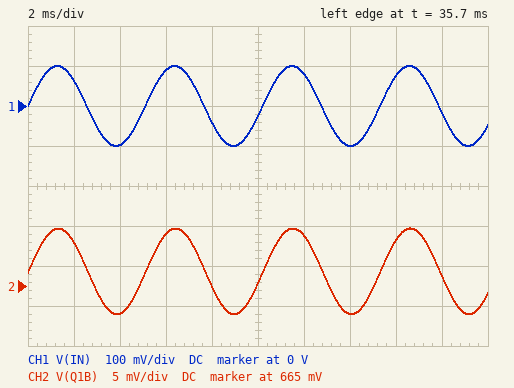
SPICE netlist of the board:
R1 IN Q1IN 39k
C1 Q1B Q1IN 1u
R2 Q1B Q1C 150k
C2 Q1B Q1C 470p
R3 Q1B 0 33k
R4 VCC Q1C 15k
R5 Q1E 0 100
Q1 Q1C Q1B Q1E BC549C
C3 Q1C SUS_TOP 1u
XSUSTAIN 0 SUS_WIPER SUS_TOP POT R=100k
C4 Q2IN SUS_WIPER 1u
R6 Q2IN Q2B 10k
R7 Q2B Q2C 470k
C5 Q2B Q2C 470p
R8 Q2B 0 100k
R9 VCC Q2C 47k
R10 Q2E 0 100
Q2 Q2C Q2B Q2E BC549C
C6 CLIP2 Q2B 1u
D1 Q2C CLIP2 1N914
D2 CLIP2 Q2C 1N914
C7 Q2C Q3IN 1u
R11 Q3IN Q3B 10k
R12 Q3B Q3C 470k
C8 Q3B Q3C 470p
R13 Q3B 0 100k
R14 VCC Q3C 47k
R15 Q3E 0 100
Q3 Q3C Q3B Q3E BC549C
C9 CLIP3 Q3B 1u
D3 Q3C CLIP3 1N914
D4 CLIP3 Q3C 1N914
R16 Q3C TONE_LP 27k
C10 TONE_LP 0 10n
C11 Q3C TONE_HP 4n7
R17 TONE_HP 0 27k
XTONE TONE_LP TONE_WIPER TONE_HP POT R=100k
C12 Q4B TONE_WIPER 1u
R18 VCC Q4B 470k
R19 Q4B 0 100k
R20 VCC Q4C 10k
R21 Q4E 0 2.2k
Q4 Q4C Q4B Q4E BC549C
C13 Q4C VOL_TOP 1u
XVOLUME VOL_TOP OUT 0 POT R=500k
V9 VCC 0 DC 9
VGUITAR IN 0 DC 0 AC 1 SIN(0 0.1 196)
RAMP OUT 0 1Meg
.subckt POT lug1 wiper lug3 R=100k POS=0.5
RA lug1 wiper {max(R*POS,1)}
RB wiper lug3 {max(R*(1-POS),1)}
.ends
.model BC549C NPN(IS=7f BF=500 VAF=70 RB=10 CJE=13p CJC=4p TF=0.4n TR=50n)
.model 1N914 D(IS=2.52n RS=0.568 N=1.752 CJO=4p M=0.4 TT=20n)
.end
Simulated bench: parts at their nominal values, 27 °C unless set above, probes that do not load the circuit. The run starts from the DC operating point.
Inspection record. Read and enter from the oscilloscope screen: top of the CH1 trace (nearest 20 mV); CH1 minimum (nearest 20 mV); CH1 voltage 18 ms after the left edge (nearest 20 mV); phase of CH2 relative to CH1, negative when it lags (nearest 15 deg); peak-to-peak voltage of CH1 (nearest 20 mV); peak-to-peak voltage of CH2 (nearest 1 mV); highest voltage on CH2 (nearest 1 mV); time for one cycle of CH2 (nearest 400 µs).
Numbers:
100 mV
-100 mV
-20 mV
0 deg
200 mV
11 mV
672 mV
5.2 ms
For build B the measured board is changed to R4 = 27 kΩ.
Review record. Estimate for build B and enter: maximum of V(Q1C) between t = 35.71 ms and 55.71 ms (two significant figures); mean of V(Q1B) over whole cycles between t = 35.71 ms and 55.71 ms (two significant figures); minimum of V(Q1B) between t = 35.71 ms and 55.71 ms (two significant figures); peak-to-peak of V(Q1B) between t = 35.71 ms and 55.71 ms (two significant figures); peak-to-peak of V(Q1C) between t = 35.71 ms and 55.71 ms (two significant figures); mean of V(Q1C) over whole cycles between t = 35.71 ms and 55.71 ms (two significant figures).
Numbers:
3.9 V
640 mV
630 mV
10 mV
660 mV
3.6 V
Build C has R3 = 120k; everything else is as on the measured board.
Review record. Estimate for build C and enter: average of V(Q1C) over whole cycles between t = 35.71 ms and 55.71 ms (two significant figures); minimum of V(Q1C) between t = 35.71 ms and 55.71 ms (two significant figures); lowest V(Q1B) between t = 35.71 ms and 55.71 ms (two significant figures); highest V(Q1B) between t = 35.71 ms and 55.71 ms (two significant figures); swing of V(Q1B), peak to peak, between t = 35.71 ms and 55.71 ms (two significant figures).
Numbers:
1.7 V
1.4 V
690 mV
700 mV
9.8 mV
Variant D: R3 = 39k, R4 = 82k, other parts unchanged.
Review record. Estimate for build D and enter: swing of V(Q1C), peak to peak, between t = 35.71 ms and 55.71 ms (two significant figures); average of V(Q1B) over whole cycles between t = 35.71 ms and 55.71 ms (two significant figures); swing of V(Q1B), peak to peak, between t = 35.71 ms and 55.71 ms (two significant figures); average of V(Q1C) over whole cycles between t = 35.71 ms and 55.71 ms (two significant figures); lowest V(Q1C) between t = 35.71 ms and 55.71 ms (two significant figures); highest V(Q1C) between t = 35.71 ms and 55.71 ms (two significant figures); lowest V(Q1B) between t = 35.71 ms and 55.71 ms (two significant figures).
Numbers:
650 mV
600 mV
13 mV
2.9 V
2.6 V
3.2 V
590 mV
